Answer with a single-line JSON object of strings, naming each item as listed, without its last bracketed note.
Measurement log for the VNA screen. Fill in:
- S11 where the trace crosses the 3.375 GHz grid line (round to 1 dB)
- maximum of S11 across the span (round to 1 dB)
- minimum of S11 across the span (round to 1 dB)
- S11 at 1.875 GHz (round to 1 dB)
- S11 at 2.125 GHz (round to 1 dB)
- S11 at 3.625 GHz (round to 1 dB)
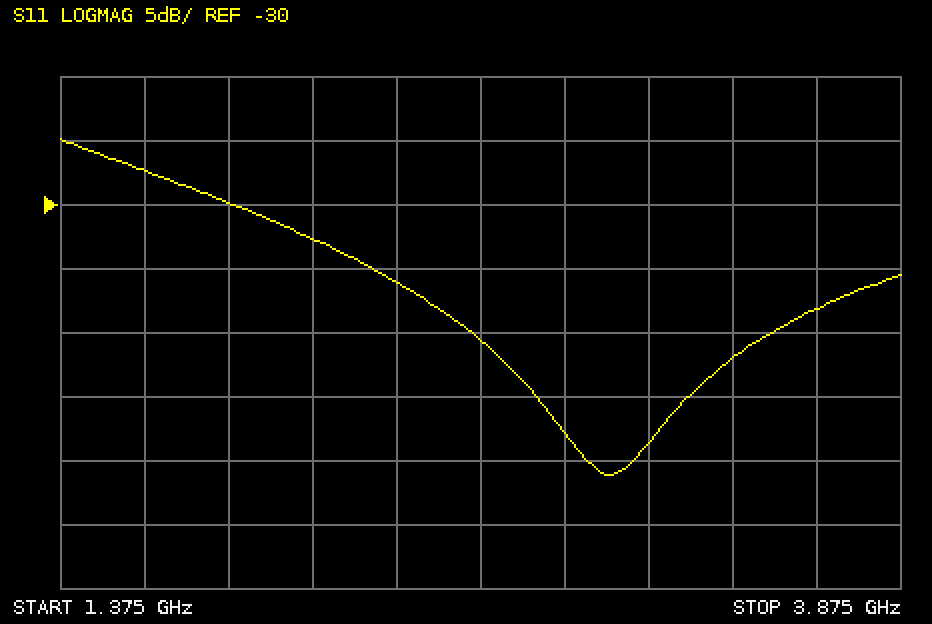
{"S11 where the trace crosses the 3.375 GHz grid line": "-42 dB", "maximum of S11 across the span": "-25 dB", "minimum of S11 across the span": "-51 dB", "S11 at 1.875 GHz": "-30 dB", "S11 at 2.125 GHz": "-33 dB", "S11 at 3.625 GHz": "-38 dB"}
